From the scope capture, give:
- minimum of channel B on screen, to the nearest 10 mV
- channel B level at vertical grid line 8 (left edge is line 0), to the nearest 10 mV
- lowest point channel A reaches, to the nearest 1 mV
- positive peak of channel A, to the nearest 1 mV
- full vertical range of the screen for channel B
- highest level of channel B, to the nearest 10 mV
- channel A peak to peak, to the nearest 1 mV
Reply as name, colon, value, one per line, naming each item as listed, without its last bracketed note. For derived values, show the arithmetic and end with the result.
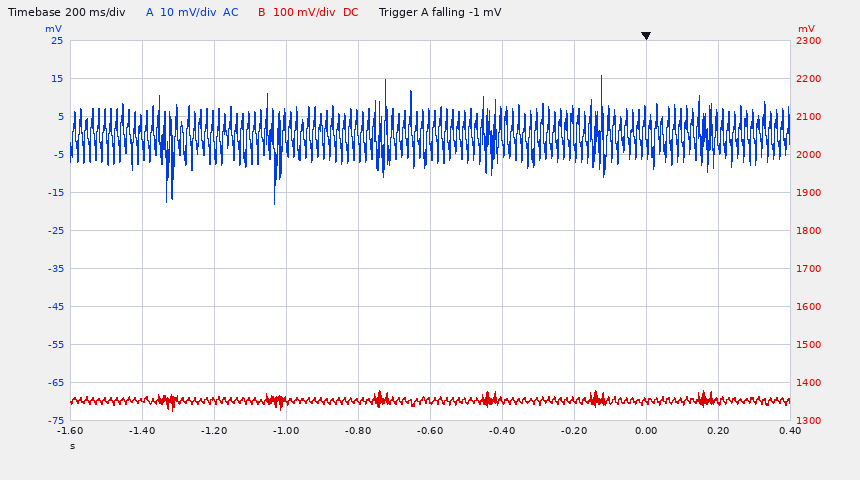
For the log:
minimum of channel B on screen, to the nearest 10 mV: 1.32 V
channel B level at vertical grid line 8 (left edge is line 0), to the nearest 10 mV: 1.35 V
lowest point channel A reaches, to the nearest 1 mV: -18 mV
positive peak of channel A, to the nearest 1 mV: 16 mV
full vertical range of the screen for channel B: 1 V
highest level of channel B, to the nearest 10 mV: 1.38 V
channel A peak to peak, to the nearest 1 mV: 16 mV − (-18 mV) = 34 mV
